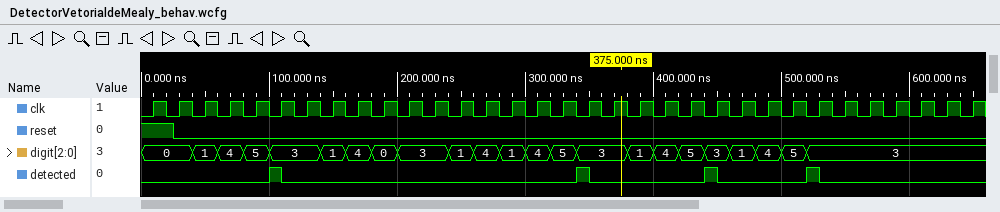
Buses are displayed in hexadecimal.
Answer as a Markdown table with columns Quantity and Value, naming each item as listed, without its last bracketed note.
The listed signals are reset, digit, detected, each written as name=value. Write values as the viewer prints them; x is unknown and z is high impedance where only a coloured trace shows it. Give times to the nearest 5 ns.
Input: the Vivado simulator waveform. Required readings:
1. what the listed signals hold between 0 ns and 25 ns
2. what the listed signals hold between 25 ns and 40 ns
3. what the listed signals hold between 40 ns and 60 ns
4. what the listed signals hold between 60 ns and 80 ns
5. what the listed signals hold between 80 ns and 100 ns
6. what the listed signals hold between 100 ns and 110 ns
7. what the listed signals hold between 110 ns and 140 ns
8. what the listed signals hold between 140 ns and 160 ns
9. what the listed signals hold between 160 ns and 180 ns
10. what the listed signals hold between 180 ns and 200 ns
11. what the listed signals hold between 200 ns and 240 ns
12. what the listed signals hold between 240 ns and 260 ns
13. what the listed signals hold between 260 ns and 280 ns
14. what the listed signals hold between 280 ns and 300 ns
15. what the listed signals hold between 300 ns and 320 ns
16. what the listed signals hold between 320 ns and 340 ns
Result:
| Quantity | Value |
|---|---|
| what the listed signals hold between 0 ns and 25 ns | reset=1, digit=0, detected=0 |
| what the listed signals hold between 25 ns and 40 ns | reset=0, digit=0, detected=0 |
| what the listed signals hold between 40 ns and 60 ns | reset=0, digit=1, detected=0 |
| what the listed signals hold between 60 ns and 80 ns | reset=0, digit=4, detected=0 |
| what the listed signals hold between 80 ns and 100 ns | reset=0, digit=5, detected=0 |
| what the listed signals hold between 100 ns and 110 ns | reset=0, digit=3, detected=1 |
| what the listed signals hold between 110 ns and 140 ns | reset=0, digit=3, detected=0 |
| what the listed signals hold between 140 ns and 160 ns | reset=0, digit=1, detected=0 |
| what the listed signals hold between 160 ns and 180 ns | reset=0, digit=4, detected=0 |
| what the listed signals hold between 180 ns and 200 ns | reset=0, digit=0, detected=0 |
| what the listed signals hold between 200 ns and 240 ns | reset=0, digit=3, detected=0 |
| what the listed signals hold between 240 ns and 260 ns | reset=0, digit=1, detected=0 |
| what the listed signals hold between 260 ns and 280 ns | reset=0, digit=4, detected=0 |
| what the listed signals hold between 280 ns and 300 ns | reset=0, digit=1, detected=0 |
| what the listed signals hold between 300 ns and 320 ns | reset=0, digit=4, detected=0 |
| what the listed signals hold between 320 ns and 340 ns | reset=0, digit=5, detected=0 |
